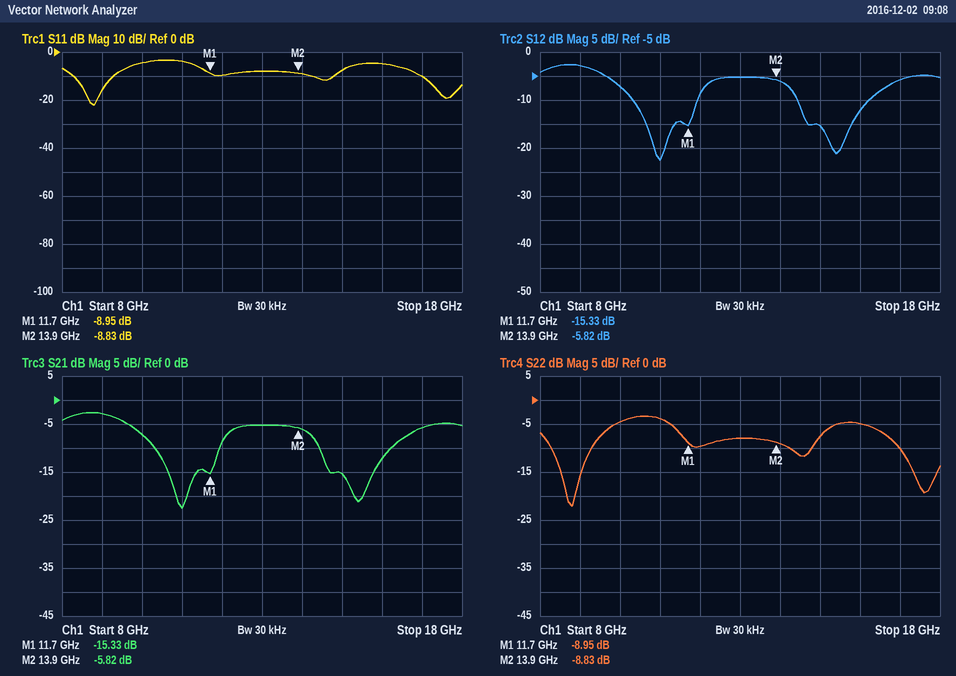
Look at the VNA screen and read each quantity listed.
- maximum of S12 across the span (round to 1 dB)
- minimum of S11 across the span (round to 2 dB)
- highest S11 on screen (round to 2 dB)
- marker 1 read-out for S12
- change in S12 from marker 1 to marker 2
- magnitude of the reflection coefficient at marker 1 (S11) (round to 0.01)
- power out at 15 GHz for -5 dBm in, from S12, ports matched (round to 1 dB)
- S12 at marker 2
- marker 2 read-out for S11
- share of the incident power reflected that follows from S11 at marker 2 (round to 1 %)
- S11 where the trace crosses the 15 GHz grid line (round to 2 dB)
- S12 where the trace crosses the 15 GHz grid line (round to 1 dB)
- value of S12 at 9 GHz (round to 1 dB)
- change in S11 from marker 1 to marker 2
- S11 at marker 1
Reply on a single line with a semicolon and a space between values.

-3 dB; -22 dB; -4 dB; -15.33 dB; 9.51 dB; 0.36; -20 dBm; -5.82 dB; -8.83 dB; 13 %; -8 dB; -15 dB; -3 dB; 0.12 dB; -8.95 dB
